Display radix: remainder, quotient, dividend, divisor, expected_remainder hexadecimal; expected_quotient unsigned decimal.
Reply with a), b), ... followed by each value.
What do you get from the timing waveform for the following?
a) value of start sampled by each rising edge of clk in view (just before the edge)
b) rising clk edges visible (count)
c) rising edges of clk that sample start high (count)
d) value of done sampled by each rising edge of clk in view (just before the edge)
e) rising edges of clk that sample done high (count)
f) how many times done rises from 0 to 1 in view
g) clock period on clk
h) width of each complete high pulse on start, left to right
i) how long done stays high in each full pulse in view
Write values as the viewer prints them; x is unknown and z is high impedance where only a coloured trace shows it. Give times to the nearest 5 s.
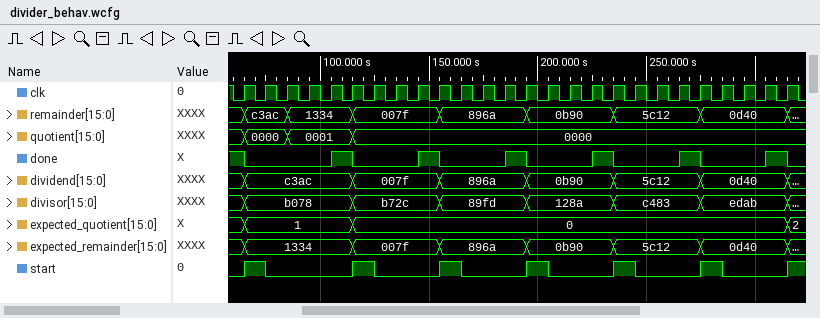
a) 0 1 0 0 0 0 1 0 0 0 1 0 0 0 1 0 0 0 1 0 0 0 1 0 0 0
b) 26
c) 6
d) 1 0 0 0 0 1 0 0 0 1 0 0 0 1 0 0 0 1 0 0 0 1 0 0 0 1
e) 7
f) 6
g) 10 s
h) 10 s, 10 s, 10 s, 10 s, 10 s, 10 s
i) 10 s, 10 s, 10 s, 10 s, 10 s, 10 s
